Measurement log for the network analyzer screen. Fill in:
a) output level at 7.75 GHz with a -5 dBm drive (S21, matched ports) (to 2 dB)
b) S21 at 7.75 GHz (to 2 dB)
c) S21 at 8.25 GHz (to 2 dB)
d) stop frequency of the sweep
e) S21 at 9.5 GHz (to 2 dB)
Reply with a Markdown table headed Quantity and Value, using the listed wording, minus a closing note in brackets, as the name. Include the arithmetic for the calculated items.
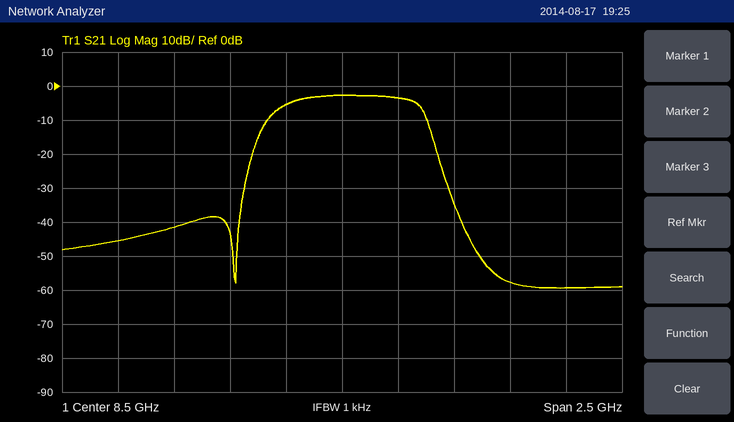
| Quantity | Value |
|---|---|
| output level at 7.75 GHz with a -5 dBm drive (S21, matched ports) | -5 dBm + (-42 dB) = -46 dBm |
| S21 at 7.75 GHz | -42 dB |
| S21 at 8.25 GHz | -6 dB |
| stop frequency of the sweep | 9.75 GHz |
| S21 at 9.5 GHz | -60 dB |
